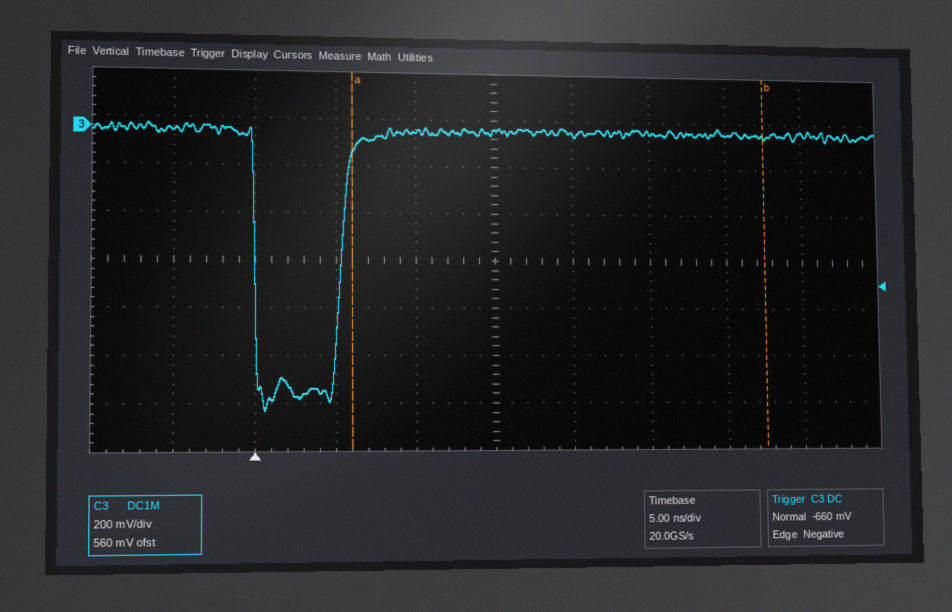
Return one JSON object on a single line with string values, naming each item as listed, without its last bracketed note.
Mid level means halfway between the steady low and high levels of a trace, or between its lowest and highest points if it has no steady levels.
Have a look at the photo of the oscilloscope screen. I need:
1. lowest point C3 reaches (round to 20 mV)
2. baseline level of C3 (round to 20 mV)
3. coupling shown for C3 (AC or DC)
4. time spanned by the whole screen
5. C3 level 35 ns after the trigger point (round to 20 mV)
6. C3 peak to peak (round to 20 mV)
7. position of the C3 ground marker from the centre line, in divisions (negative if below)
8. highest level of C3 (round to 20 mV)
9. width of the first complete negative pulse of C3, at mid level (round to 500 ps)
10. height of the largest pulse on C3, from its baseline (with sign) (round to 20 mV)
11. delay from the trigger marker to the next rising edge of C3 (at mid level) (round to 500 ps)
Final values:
{"lowest point C3 reaches": "-1.18 V", "baseline level of C3": "0 mV", "coupling shown for C3": "DC", "time spanned by the whole screen": "50 ns", "C3 level 35 ns after the trigger point": "0 mV", "C3 peak to peak": "1.20 V", "position of the C3 ground marker from the centre line, in divisions": "+2.8 div", "highest level of C3": "20 mV", "width of the first complete negative pulse of C3, at mid level": "5.5 ns", "height of the largest pulse on C3, from its baseline (with sign)": "-1.18 V", "delay from the trigger marker to the next rising edge of C3 (at mid level)": "5.5 ns"}
